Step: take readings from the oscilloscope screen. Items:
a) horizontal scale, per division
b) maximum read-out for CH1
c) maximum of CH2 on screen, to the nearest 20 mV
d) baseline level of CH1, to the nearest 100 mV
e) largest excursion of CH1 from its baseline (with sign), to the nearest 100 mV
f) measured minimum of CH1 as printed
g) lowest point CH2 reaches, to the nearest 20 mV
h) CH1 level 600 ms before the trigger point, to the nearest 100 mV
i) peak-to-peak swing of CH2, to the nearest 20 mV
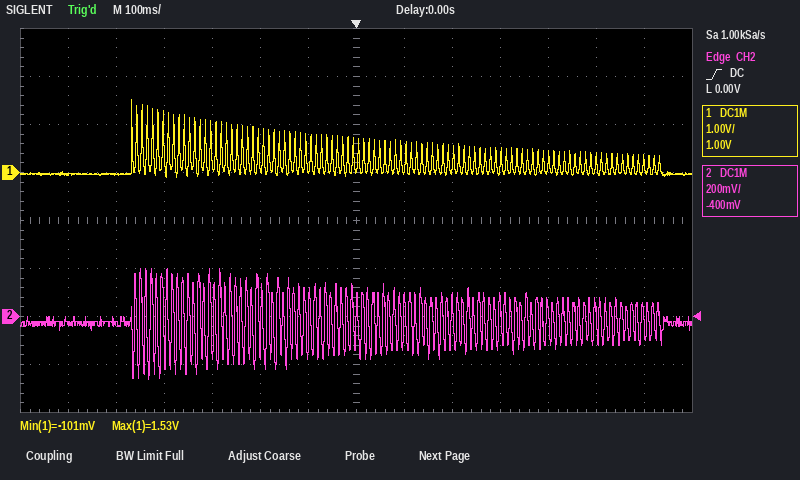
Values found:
100 ms
1.53 V
200 mV
0.0 V
+1.5 V
-101 mV
-260 mV
0.0 V
460 mV
